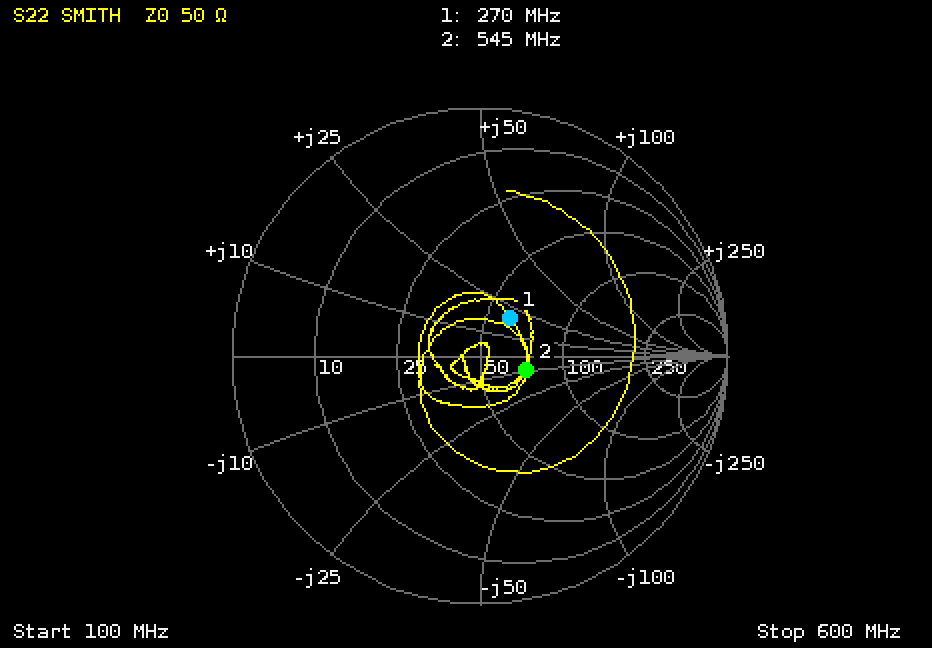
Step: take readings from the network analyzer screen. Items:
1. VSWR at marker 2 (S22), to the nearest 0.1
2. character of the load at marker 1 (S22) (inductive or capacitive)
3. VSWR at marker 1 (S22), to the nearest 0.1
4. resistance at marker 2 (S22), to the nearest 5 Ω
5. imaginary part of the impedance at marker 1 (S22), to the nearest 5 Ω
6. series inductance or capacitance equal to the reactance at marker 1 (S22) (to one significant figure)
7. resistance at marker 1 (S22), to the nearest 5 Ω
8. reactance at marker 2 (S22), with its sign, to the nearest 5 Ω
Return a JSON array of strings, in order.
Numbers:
["1.5", "inductive", "1.5", "70 Ω", "+20 Ω", "10 nH", "60 Ω", "-10 Ω"]
